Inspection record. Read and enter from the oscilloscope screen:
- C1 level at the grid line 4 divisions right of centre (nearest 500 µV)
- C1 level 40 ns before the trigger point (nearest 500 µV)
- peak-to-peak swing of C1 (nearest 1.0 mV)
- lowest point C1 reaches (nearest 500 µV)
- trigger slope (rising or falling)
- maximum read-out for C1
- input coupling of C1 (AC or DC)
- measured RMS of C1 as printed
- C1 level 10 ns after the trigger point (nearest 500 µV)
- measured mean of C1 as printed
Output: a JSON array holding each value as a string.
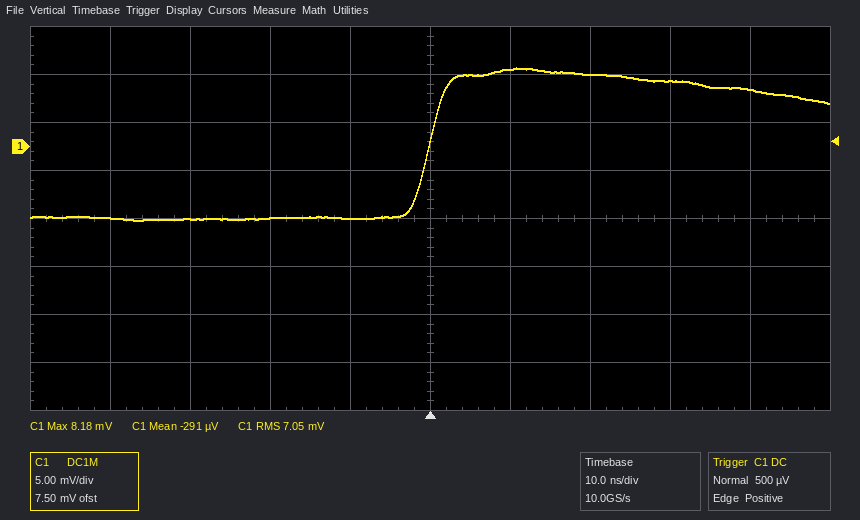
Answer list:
["6.0 mV", "-7.5 mV", "16.0 mV", "-7.5 mV", "rising", "8.18 mV", "DC", "7.05 mV", "8.0 mV", "-291 µV"]
